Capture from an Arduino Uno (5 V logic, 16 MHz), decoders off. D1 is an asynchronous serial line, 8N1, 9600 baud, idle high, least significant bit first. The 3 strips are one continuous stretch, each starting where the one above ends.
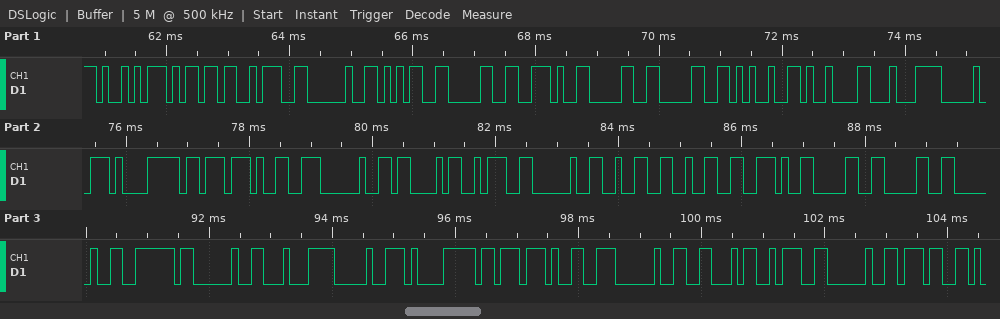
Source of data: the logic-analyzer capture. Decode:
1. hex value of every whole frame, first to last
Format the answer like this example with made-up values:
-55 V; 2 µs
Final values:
A9 6D 3A 20 35 30 2E 30 30 25 09 C4 90 E1 BB 99 20 43 3A 20 32 32 2E 30 30 20 7E 20 C4 90 E1 BB 99 20 46 3A 20 37
